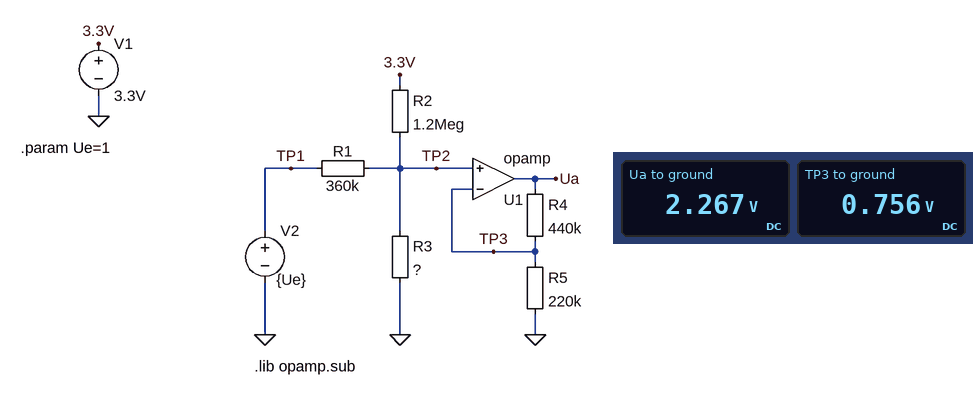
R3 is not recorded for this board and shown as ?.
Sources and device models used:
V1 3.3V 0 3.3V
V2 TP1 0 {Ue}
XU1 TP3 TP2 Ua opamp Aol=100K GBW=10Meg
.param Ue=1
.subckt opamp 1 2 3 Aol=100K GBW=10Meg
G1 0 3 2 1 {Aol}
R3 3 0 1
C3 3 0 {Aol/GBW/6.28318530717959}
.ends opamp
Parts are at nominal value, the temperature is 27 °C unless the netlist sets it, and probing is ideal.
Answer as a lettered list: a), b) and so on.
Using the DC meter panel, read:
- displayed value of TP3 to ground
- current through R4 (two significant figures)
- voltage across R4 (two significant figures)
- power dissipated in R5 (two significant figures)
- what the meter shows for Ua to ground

a) 0.756 V
b) 3.4 µA
c) 1.5 V
d) 2.6 µW
e) 2.267 V
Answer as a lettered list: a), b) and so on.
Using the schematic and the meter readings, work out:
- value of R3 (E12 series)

a) 270 kΩ
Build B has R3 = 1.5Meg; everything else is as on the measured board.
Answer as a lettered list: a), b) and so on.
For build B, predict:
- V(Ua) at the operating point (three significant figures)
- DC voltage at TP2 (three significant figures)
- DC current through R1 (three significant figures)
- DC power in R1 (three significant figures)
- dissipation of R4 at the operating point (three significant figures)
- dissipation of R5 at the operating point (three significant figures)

a) 3.88 V
b) 1.29 V
c) 812 nA
d) 237 nW
e) 15.2 µW
f) 7.59 µW
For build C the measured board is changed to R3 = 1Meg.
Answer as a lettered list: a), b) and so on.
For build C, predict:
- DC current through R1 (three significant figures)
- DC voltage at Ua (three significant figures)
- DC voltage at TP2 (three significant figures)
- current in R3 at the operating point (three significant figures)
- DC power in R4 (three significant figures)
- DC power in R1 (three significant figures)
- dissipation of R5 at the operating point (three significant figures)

a) 552 nA
b) 3.60 V
c) 1.20 V
d) 1.20 µA
e) 13.1 µW
f) 110 nW
g) 6.53 µW
